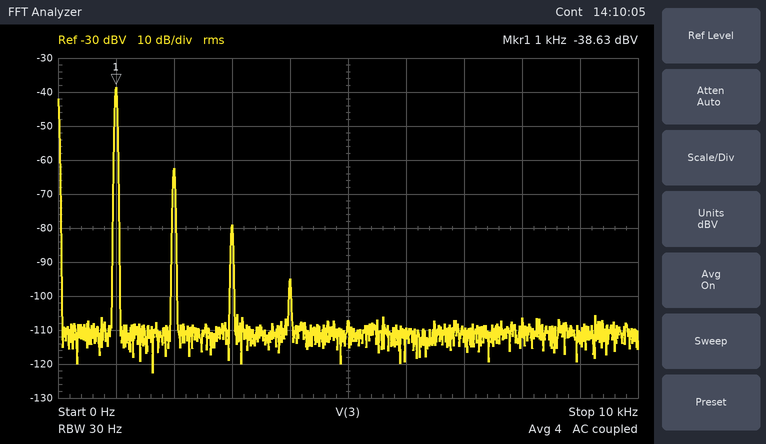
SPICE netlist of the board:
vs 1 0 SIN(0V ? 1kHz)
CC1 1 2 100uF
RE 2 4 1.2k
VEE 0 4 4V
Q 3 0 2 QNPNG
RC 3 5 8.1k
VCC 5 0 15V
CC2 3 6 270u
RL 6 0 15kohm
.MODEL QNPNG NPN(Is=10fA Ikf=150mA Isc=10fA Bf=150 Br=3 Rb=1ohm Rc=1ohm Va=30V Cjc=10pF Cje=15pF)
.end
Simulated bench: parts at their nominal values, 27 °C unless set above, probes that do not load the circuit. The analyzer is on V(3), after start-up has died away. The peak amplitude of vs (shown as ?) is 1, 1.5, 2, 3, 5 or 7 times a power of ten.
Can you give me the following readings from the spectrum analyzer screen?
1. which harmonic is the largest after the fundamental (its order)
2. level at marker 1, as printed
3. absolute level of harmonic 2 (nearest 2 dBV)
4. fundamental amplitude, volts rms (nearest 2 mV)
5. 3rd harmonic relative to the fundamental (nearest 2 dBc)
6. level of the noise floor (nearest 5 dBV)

2
-38.63 dBV
-62 dBV
12 mV
-40 dBc
-110 dBV
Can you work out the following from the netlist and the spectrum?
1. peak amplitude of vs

10 mV
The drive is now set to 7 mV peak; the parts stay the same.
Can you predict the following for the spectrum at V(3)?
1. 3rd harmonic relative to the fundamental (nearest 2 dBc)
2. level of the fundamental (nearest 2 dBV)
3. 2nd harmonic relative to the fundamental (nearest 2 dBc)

-48 dBc
-42 dBV
-28 dBc
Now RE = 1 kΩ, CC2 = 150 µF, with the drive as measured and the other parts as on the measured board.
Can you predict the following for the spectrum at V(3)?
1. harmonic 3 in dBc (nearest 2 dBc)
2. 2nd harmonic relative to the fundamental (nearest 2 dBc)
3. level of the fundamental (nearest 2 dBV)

-48 dBc
-28 dBc
-40 dBV
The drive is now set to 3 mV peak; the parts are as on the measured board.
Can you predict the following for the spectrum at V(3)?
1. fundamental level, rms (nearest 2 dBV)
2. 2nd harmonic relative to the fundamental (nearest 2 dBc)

-50 dBV
-36 dBc
